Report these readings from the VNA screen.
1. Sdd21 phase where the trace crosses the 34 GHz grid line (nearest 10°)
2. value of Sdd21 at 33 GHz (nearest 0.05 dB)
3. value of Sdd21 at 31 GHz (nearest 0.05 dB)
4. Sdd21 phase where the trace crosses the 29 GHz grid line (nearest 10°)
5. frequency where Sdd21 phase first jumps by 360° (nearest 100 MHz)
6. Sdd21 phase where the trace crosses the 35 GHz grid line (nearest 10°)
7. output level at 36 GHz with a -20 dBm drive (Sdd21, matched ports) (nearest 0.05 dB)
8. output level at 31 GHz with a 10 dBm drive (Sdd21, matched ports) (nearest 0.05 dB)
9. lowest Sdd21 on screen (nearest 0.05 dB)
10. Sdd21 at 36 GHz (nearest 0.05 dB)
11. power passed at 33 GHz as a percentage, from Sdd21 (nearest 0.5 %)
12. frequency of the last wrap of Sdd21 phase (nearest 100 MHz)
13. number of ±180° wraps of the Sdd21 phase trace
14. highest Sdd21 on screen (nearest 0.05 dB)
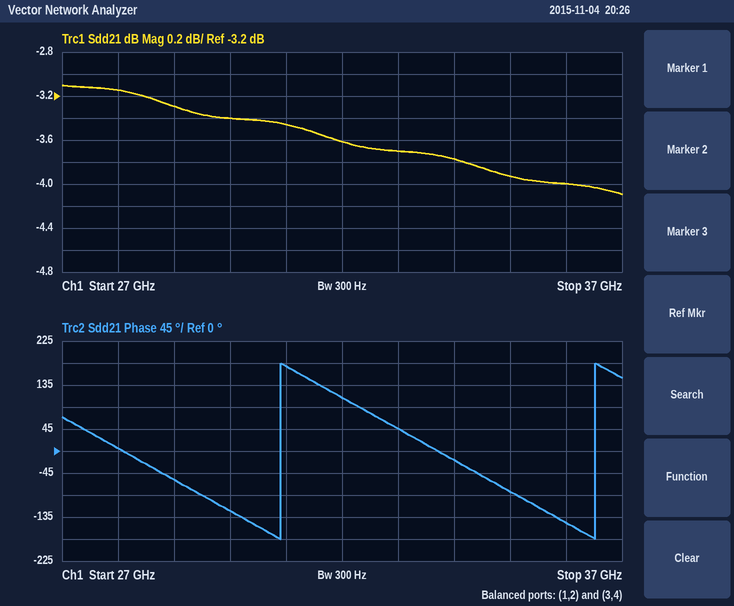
-20°
-3.70 dB
-3.45 dB
-60°
30.9 GHz
-80°
-24.00 dBm
6.55 dBm
-4.10 dB
-4.00 dB
42.5 %
36.5 GHz
2
-3.10 dB
